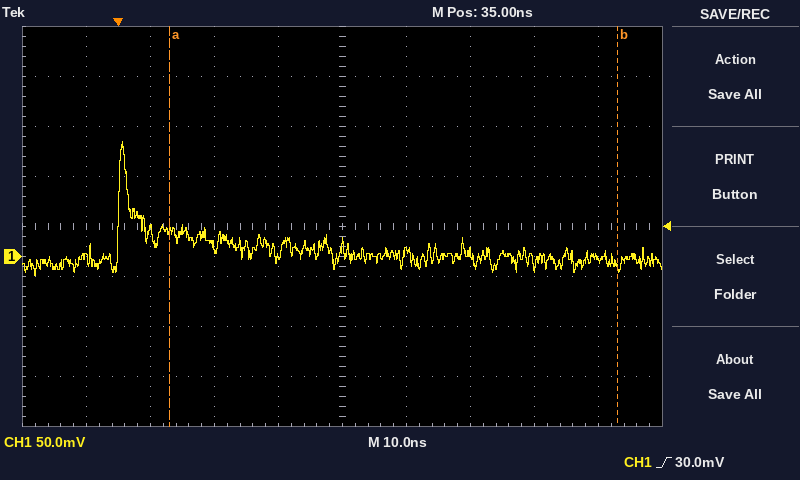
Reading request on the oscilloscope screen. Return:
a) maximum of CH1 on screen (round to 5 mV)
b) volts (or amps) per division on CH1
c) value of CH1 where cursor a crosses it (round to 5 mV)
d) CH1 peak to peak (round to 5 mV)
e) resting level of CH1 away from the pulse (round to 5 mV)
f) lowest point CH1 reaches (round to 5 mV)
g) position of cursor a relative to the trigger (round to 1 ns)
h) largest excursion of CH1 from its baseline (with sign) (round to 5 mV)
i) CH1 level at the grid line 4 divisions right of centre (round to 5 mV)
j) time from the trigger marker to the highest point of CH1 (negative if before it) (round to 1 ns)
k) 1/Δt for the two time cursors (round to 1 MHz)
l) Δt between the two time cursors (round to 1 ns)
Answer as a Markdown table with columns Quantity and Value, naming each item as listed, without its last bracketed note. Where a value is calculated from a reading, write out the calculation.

| Quantity | Value |
|---|---|
| maximum of CH1 on screen | 115 mV |
| volts (or amps) per division on CH1 | 50 mV |
| value of CH1 where cursor a crosses it | 25 mV |
| CH1 peak to peak | 115 mV − (-20 mV) = 135 mV |
| resting level of CH1 away from the pulse | 0 mV |
| lowest point CH1 reaches | -20 mV |
| position of cursor a relative to the trigger | +8 ns |
| largest excursion of CH1 from its baseline (with sign) | 115 mV − (0 mV) = +115 mV |
| CH1 level at the grid line 4 divisions right of centre | 0 mV |
| time from the trigger marker to the highest point of CH1 (negative if before it) | +1 ns |
| 1/Δt for the two time cursors | 1 / 70 ns ≈ 14 MHz |
| Δt between the two time cursors | 70 ns |
